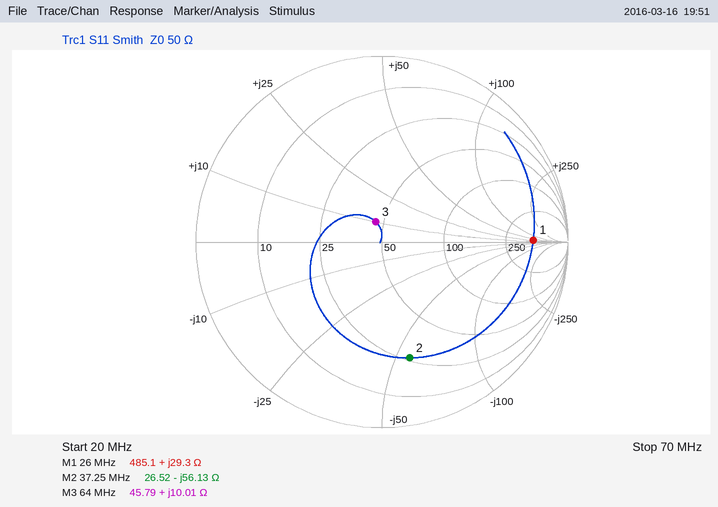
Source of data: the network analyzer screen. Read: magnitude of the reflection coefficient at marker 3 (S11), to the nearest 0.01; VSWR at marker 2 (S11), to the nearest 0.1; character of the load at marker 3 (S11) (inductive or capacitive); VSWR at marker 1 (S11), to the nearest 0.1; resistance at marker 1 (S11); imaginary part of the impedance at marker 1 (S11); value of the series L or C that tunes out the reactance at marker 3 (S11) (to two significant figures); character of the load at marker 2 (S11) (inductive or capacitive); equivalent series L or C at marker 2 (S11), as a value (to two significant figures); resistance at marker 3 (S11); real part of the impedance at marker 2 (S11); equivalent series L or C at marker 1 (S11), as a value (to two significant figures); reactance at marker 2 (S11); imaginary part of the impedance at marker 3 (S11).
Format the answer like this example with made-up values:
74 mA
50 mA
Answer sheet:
0.11
4.6
inductive
9.7
485.1 Ω
+29.3 Ω
250 pF
capacitive
76 pF
45.79 Ω
26.52 Ω
180 nH
-56.13 Ω
+10.01 Ω
